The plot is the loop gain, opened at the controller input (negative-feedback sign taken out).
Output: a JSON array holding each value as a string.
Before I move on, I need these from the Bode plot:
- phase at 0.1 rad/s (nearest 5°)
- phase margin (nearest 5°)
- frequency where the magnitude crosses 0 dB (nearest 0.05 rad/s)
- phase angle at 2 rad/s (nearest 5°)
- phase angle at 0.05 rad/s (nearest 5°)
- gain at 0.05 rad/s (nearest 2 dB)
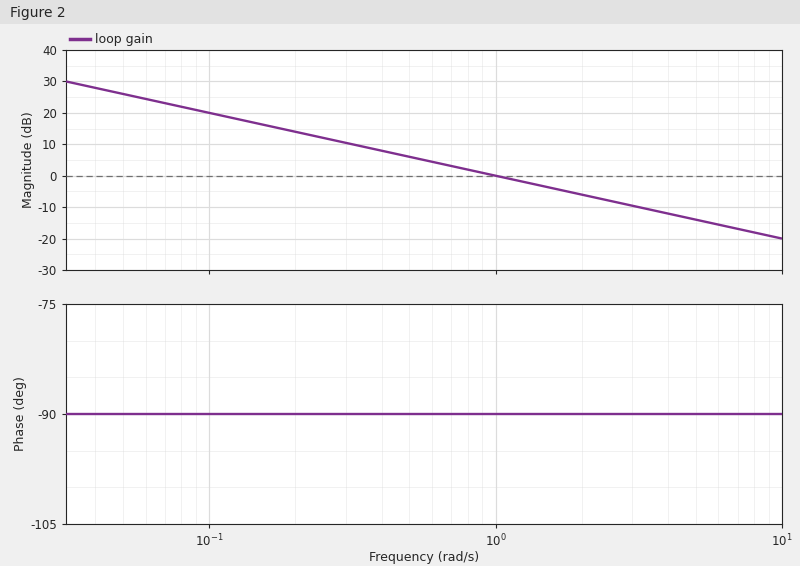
["-90°", "90°", "1.00 rad/s", "-90°", "-90°", "26 dB"]
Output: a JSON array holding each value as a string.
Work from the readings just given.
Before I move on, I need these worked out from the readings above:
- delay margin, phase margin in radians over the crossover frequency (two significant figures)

["1.6 s"]
